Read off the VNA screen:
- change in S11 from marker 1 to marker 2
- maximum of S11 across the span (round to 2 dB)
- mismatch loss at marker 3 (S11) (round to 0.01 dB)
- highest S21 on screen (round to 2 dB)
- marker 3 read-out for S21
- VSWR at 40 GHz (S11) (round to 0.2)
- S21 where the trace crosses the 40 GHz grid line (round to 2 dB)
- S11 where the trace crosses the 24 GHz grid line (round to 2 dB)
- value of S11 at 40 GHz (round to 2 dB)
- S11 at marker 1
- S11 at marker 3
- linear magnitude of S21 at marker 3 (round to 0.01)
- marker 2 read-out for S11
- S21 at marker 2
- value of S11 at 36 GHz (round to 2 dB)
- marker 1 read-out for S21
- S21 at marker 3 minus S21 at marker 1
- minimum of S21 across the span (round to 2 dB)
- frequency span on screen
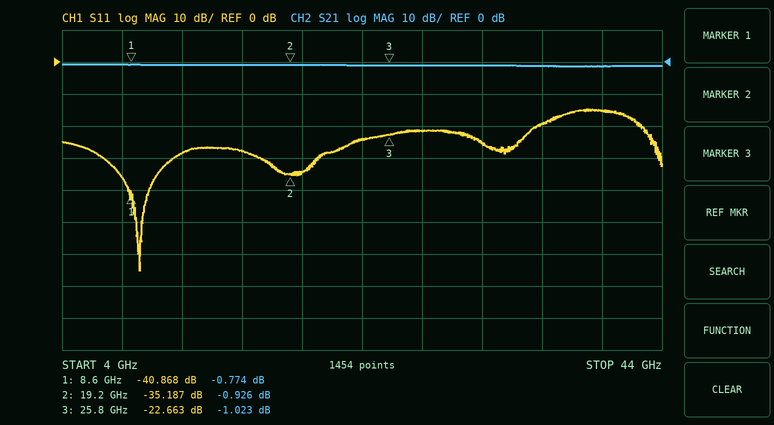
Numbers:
5.681 dB
-14 dB
0.02 dB
0 dB
-1.023 dB
1.4
-2 dB
-24 dB
-16 dB
-40.868 dB
-22.663 dB
0.89
-35.187 dB
-0.926 dB
-20 dB
-0.774 dB
-0.249 dB
-2 dB
40 GHz
